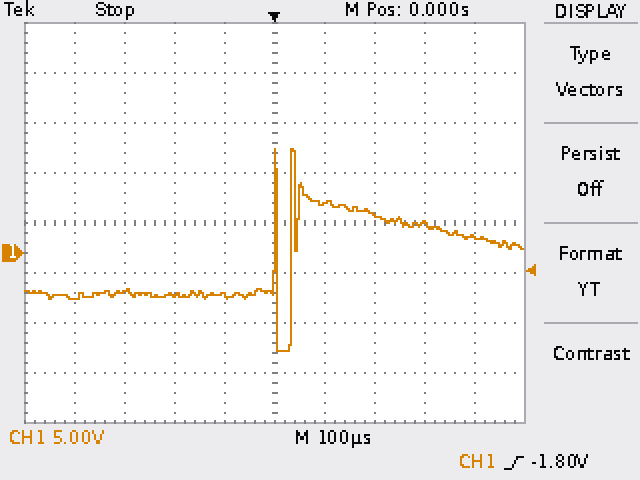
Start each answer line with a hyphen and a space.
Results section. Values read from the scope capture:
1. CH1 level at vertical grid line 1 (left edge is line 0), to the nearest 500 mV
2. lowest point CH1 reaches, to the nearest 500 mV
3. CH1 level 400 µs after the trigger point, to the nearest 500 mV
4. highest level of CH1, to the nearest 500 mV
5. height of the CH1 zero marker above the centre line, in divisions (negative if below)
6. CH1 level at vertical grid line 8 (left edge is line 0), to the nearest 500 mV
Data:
- -4.5 V
- -10.0 V
- 1.5 V
- 10.5 V
- -0.6 div
- 3.0 V
